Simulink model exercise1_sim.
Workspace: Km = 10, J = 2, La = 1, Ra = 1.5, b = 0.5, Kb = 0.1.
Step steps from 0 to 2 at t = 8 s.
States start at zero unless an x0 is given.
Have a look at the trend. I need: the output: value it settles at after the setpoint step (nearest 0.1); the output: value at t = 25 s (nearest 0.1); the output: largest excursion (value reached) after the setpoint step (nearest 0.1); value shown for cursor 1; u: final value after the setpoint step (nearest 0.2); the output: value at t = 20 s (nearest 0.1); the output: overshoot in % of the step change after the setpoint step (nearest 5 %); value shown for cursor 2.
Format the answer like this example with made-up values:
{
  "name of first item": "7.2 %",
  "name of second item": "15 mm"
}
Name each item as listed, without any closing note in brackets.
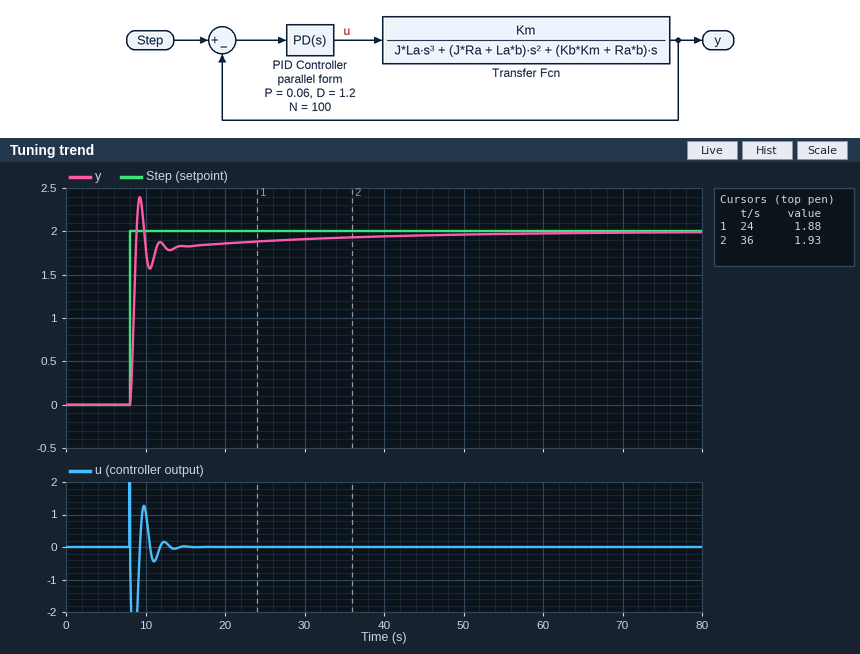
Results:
{
  "the output: value it settles at after the setpoint step": "2.0",
  "the output: value at t = 25 s": "1.9",
  "the output: largest excursion (value reached) after the setpoint step": "2.4",
  "value shown for cursor 1": "1.88",
  "u: final value after the setpoint step": "0.0",
  "the output: value at t = 20 s": "1.9",
  "the output: overshoot in % of the step change after the setpoint step": "20 %",
  "value shown for cursor 2": "1.93"
}
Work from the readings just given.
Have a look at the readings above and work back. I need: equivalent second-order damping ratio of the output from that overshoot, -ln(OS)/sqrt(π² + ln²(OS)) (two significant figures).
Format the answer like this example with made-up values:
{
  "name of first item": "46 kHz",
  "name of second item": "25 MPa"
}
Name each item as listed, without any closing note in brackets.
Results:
{
  "equivalent second-order damping ratio of the output from that overshoot, -ln(OS)/sqrt(π² + ln²(OS))": "0.46"
}
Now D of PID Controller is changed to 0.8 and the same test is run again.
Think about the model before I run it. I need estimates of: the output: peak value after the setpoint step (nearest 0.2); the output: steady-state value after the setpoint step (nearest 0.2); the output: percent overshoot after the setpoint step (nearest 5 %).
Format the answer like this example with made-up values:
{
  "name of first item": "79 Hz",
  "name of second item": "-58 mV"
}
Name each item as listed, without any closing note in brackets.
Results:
{
  "the output: peak value after the setpoint step": "2.2",
  "the output: steady-state value after the setpoint step": "2.0",
  "the output: percent overshoot after the setpoint step": "10 %"
}
